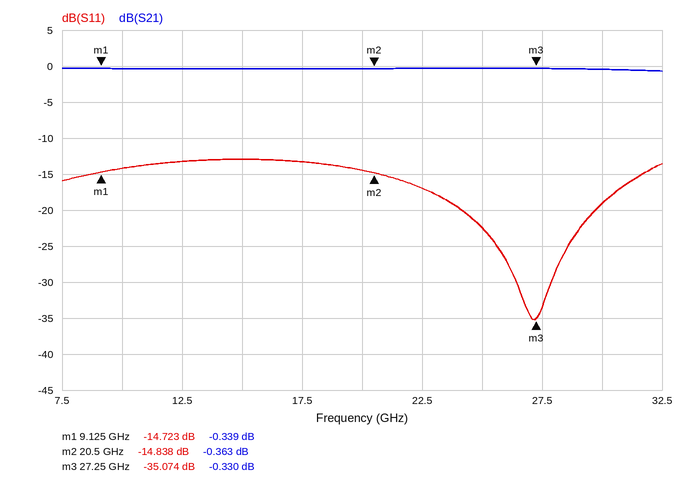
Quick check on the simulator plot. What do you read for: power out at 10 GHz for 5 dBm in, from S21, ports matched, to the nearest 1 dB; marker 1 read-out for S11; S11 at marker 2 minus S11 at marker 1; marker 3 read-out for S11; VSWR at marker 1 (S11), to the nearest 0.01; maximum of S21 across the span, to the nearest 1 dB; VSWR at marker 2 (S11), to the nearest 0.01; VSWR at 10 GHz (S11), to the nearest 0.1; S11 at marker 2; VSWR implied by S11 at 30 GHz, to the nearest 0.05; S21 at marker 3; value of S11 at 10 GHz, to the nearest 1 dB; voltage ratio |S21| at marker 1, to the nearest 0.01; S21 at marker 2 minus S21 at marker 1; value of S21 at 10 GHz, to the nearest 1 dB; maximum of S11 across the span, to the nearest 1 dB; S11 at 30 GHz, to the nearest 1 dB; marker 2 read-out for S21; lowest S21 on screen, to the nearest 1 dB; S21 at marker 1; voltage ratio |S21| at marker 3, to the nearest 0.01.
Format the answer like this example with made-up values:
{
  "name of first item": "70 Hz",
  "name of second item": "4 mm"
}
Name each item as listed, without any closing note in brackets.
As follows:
{
  "power out at 10 GHz for 5 dBm in, from S21, ports matched, to the nearest 1 dB": "5 dBm",
  "marker 1 read-out for S11": "-14.723 dB",
  "S11 at marker 2 minus S11 at marker 1": "-0.115 dB",
  "marker 3 read-out for S11": "-35.074 dB",
  "VSWR at marker 1 (S11), to the nearest 0.01": "1.45",
  "maximum of S21 across the span, to the nearest 1 dB": "0 dB",
  "VSWR at marker 2 (S11), to the nearest 0.01": "1.44",
  "VSWR at 10 GHz (S11), to the nearest 0.1": "1.5",
  "S11 at marker 2": "-14.838 dB",
  "VSWR implied by S11 at 30 GHz, to the nearest 0.05": "1.25",
  "S21 at marker 3": "-0.330 dB",
  "value of S11 at 10 GHz, to the nearest 1 dB": "-14 dB",
  "voltage ratio |S21| at marker 1, to the nearest 0.01": "0.96",
  "S21 at marker 2 minus S21 at marker 1": "-0.024 dB",
  "value of S21 at 10 GHz, to the nearest 1 dB": "0 dB",
  "maximum of S11 across the span, to the nearest 1 dB": "-13 dB",
  "S11 at 30 GHz, to the nearest 1 dB": "-19 dB",
  "marker 2 read-out for S21": "-0.363 dB",
  "lowest S21 on screen, to the nearest 1 dB": "-1 dB",
  "S21 at marker 1": "-0.339 dB",
  "voltage ratio |S21| at marker 3, to the nearest 0.01": "0.96"
}
